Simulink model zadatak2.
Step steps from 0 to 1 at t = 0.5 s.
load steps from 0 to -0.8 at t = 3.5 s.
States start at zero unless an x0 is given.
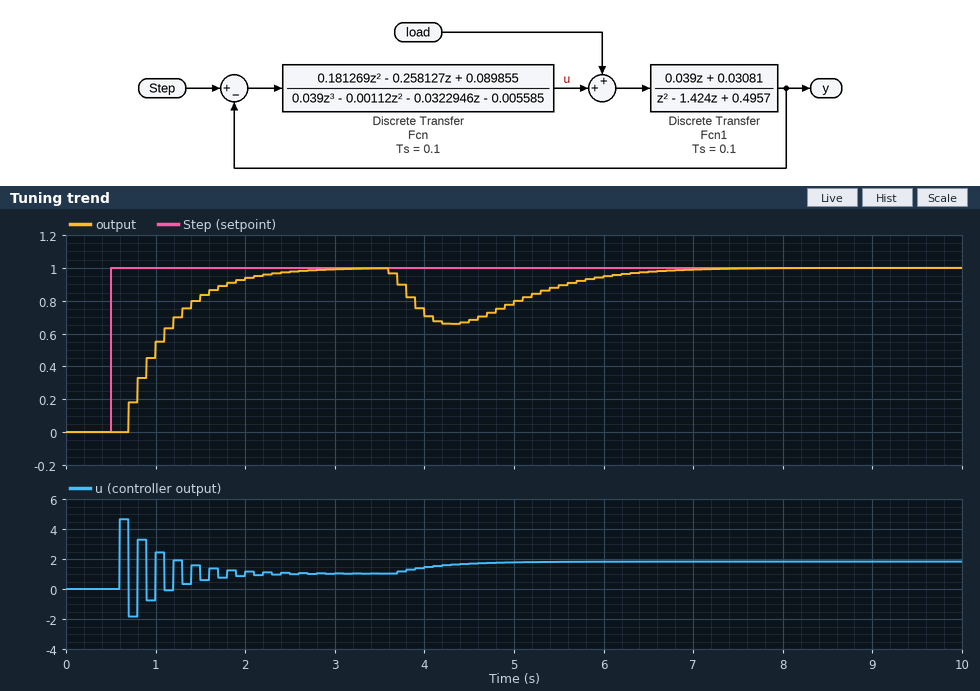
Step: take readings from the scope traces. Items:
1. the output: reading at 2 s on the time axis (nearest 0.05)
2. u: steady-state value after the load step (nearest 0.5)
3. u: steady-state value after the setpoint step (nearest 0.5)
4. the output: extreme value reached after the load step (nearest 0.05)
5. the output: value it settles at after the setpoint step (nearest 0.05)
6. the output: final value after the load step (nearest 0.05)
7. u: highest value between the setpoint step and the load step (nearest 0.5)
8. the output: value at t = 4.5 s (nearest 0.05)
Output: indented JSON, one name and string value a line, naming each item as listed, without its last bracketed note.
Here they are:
{
  "the output: reading at 2 s on the time axis": "0.95",
  "u: steady-state value after the load step": "2.0",
  "u: steady-state value after the setpoint step": "1.0",
  "the output: extreme value reached after the load step": "0.65",
  "the output: value it settles at after the setpoint step": "1.00",
  "the output: final value after the load step": "1.00",
  "u: highest value between the setpoint step and the load step": "4.5",
  "the output: value at t = 4.5 s": "0.70"
}
